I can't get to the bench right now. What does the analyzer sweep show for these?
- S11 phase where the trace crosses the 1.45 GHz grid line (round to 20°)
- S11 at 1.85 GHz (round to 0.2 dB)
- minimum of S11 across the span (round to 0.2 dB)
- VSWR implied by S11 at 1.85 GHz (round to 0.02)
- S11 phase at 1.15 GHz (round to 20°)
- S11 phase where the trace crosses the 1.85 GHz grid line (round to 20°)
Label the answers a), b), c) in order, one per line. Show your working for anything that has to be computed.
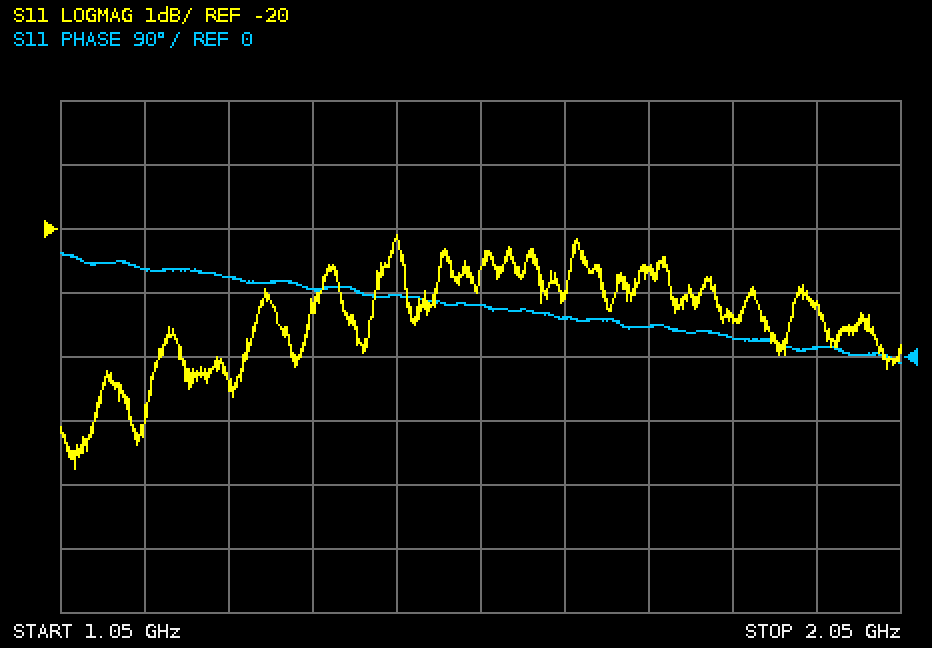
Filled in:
a) 80°
b) -21.4 dB
c) -23.8 dB
d) |Γ| = 10^(-21.4/20) = 0.0851; VSWR = (1 + 0.0851)/(1 − 0.0851) ≈ 1.19, so 1.18 to the nearest 0.02
e) 120°
f) 20°
